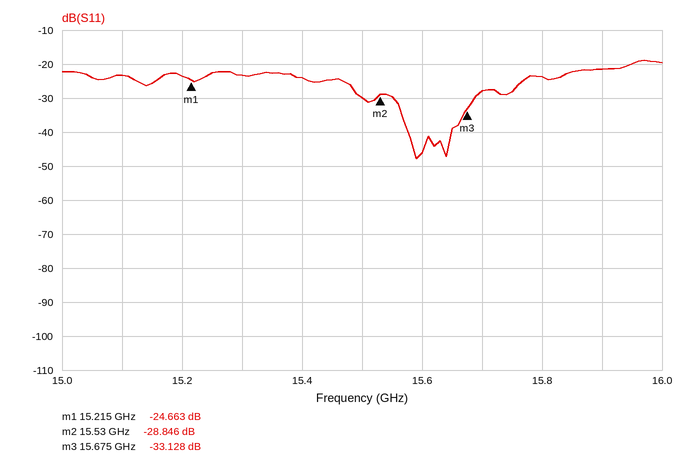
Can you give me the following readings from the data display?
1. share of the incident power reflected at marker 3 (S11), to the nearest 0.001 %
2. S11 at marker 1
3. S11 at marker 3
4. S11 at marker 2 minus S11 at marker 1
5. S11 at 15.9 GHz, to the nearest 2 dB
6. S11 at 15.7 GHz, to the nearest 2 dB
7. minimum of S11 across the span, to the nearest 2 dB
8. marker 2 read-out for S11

0.049 %
-24.663 dB
-33.128 dB
-4.183 dB
-22 dB
-28 dB
-48 dB
-28.846 dB
